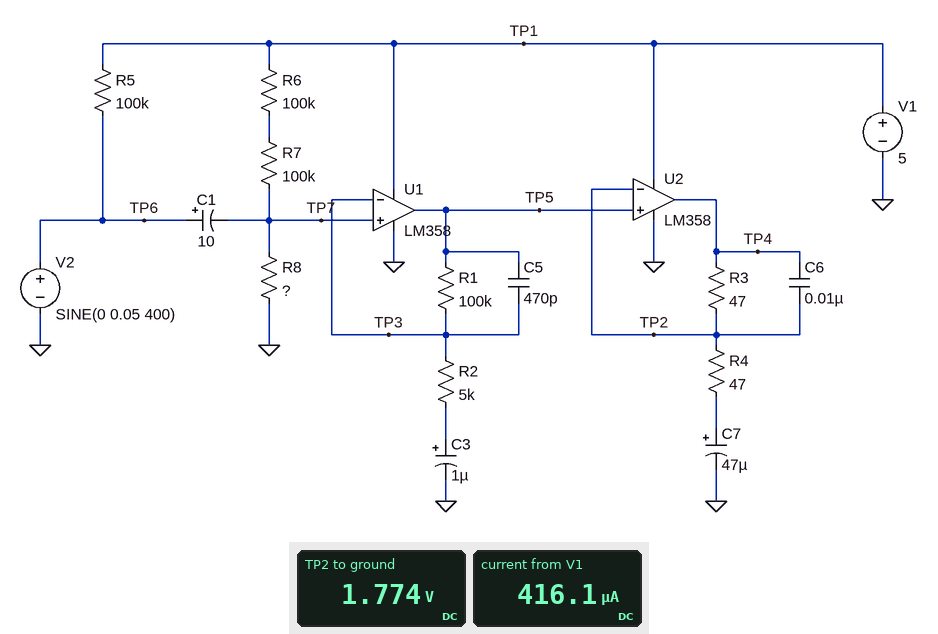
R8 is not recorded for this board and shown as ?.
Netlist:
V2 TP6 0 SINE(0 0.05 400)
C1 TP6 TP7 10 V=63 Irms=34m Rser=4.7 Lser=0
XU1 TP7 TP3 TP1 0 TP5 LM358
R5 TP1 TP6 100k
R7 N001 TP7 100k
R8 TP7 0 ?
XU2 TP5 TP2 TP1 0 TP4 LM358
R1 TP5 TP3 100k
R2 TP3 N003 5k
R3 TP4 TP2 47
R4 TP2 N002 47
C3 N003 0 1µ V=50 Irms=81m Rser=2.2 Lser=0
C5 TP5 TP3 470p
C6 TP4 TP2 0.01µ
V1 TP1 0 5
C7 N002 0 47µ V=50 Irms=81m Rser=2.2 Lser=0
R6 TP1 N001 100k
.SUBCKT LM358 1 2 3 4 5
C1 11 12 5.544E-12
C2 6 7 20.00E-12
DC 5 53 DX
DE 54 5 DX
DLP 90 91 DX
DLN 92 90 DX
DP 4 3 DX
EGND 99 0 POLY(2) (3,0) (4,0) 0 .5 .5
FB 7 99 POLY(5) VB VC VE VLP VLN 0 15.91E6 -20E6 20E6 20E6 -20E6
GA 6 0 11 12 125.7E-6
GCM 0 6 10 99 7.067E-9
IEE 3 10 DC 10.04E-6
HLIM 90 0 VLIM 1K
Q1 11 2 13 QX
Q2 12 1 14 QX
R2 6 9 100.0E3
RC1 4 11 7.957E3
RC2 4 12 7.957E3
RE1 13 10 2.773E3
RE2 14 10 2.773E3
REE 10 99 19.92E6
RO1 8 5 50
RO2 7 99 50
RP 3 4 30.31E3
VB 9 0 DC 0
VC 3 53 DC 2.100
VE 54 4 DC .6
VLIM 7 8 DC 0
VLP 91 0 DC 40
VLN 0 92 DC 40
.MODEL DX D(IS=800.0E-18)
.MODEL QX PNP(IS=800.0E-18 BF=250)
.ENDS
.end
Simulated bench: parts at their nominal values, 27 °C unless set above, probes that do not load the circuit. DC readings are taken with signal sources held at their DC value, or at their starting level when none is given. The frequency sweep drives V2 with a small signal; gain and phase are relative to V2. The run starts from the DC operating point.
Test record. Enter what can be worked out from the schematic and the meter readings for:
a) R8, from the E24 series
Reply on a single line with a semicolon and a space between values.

110 kΩ
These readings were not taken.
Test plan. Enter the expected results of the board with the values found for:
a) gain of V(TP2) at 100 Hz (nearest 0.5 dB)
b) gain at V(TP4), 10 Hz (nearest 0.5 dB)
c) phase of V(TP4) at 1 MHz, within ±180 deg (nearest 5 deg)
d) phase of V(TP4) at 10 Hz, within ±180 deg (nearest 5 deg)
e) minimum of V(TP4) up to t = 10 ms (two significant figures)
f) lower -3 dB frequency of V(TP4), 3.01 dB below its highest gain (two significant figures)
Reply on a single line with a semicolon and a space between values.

26.0 dB; 16.5 dB; -170 deg; 70 deg; 4.5 mV; 63 Hz
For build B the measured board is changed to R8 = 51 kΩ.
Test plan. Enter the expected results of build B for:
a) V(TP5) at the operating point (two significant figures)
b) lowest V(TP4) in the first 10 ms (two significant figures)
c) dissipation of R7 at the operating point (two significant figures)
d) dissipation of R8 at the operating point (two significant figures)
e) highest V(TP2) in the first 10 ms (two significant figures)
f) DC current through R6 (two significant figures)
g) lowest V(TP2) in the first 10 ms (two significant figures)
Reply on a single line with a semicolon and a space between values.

1.0 V; 4.4 mV; 40 µW; 20 µW; 2.0 V; 20 µA; 500 mV
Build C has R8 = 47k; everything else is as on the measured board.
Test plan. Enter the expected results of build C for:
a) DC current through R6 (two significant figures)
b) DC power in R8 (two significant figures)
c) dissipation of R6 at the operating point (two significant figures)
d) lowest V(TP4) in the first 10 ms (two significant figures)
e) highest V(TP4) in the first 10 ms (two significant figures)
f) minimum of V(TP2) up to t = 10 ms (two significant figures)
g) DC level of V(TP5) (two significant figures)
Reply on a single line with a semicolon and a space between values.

20 µA; 19 µW; 41 µW; 4.4 mV; 2.8 V; 470 mV; 950 mV
